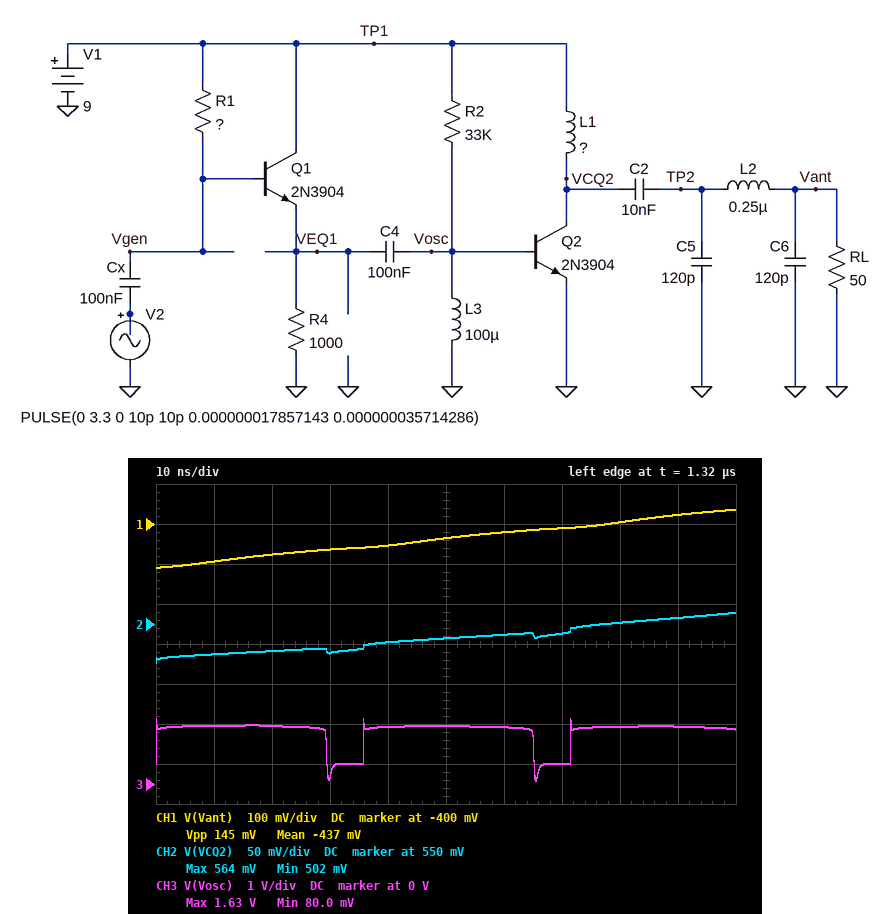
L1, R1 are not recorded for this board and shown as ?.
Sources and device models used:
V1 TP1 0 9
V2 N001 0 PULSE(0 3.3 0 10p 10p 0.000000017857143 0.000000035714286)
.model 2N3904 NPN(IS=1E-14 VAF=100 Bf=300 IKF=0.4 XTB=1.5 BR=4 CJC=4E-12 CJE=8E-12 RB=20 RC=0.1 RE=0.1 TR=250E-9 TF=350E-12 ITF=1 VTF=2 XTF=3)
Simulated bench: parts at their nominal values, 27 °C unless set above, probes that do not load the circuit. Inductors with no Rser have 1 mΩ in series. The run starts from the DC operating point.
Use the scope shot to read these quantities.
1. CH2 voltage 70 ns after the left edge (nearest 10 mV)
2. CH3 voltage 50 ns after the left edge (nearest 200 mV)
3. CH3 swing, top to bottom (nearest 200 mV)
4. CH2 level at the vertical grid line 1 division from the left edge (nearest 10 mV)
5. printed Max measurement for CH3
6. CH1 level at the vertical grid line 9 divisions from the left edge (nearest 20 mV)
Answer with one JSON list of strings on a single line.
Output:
["540 mV", "1.4 V", "1.6 V", "510 mV", "1.63 V", "-380 mV"]
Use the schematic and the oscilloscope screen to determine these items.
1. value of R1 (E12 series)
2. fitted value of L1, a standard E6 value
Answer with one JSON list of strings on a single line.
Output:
["56 kΩ", "6.8 µH"]
